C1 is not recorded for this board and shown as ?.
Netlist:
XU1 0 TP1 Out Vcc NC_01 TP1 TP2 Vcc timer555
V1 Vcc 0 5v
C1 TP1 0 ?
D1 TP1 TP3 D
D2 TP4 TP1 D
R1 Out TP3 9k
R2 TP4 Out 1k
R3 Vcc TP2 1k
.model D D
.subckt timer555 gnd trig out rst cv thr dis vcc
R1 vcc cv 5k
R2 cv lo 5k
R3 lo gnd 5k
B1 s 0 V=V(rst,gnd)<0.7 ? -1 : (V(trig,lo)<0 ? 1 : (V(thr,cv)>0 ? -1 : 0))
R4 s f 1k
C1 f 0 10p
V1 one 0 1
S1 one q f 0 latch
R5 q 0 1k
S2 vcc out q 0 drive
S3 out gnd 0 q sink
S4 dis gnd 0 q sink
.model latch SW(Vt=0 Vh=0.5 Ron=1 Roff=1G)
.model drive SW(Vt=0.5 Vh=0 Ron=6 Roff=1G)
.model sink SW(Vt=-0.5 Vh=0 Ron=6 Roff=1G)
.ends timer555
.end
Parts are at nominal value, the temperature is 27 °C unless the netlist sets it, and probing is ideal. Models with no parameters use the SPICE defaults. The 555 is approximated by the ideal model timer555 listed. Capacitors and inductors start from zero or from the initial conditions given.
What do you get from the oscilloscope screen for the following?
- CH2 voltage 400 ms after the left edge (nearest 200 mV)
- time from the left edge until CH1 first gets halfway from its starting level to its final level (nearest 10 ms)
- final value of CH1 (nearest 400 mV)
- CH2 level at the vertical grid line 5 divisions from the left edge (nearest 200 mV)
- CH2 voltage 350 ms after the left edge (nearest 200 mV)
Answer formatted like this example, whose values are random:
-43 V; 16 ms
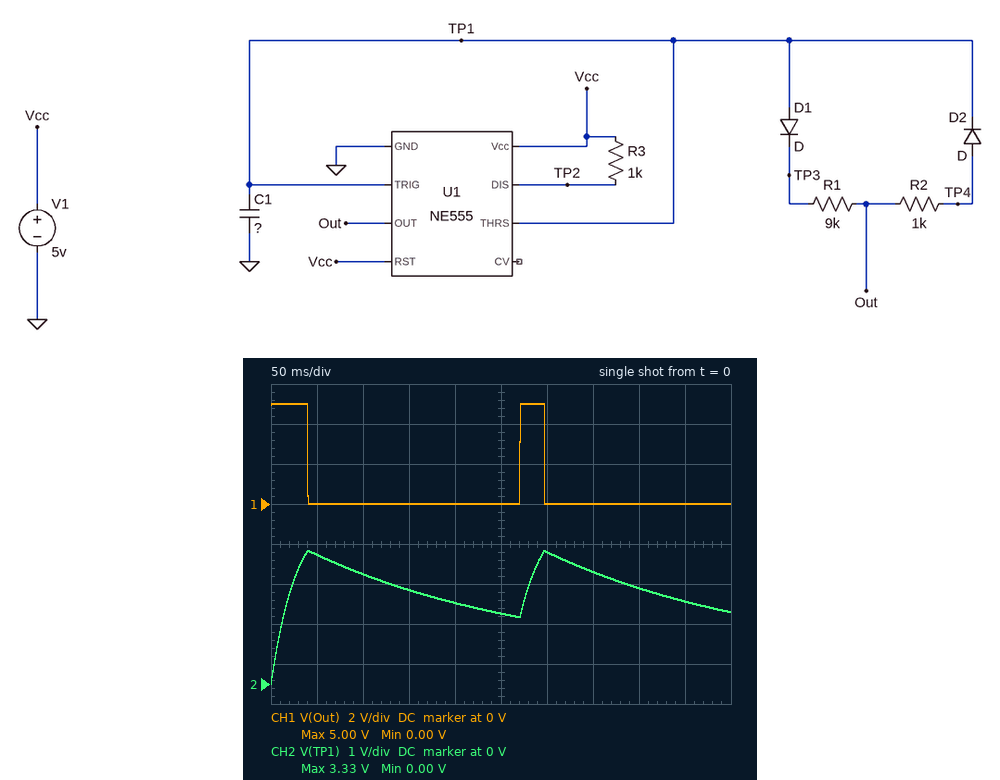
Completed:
2.4 V; 40 ms; 0 V; 1.8 V; 2.8 V
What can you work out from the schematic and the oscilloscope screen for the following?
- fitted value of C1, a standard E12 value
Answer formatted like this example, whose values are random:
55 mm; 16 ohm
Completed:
27 µF
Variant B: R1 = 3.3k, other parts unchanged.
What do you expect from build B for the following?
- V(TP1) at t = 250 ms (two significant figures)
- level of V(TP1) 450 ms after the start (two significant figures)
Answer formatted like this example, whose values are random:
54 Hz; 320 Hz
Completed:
2.6 V; 1.8 V
